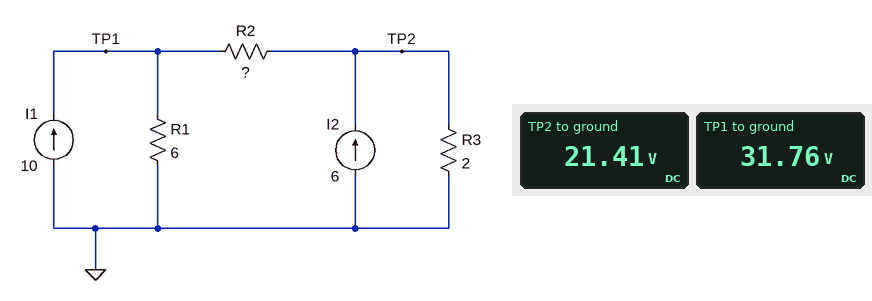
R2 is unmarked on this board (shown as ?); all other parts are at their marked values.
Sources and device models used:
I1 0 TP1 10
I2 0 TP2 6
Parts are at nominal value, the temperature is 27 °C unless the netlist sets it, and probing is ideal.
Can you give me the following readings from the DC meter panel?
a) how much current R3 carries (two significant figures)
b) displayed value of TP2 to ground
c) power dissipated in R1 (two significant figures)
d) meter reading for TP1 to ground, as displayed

11 A
21.41 V
170 W
31.76 V
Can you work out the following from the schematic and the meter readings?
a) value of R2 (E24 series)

2.2 Ω
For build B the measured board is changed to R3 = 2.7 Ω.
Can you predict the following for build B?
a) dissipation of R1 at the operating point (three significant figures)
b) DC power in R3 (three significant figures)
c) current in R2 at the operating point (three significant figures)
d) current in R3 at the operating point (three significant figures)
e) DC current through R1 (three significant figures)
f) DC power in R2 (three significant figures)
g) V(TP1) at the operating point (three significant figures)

215 W
271 W
4.02 A
10.0 A
5.98 A
35.5 W
35.9 V
